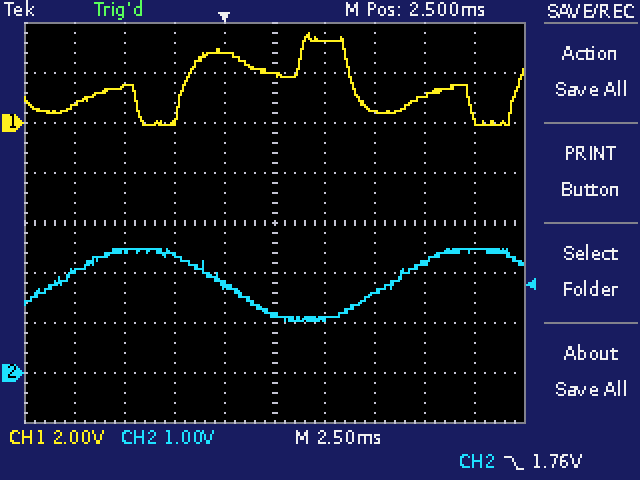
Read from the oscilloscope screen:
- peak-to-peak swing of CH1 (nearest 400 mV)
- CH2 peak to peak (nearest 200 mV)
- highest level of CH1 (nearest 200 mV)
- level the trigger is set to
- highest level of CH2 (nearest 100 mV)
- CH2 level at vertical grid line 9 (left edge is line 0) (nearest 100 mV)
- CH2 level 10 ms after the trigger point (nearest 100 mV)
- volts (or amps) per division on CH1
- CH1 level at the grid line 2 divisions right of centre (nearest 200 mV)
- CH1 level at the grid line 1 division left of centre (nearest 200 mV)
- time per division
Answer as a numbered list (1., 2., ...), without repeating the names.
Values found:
1. 3.6 V
2. 1.4 V
3. 3.6 V
4. 1.76 V
5. 2.5 V
6. 2.5 V
7. 2.2 V
8. 2 V
9. 400 mV
10. 2.8 V
11. 2.5 ms
